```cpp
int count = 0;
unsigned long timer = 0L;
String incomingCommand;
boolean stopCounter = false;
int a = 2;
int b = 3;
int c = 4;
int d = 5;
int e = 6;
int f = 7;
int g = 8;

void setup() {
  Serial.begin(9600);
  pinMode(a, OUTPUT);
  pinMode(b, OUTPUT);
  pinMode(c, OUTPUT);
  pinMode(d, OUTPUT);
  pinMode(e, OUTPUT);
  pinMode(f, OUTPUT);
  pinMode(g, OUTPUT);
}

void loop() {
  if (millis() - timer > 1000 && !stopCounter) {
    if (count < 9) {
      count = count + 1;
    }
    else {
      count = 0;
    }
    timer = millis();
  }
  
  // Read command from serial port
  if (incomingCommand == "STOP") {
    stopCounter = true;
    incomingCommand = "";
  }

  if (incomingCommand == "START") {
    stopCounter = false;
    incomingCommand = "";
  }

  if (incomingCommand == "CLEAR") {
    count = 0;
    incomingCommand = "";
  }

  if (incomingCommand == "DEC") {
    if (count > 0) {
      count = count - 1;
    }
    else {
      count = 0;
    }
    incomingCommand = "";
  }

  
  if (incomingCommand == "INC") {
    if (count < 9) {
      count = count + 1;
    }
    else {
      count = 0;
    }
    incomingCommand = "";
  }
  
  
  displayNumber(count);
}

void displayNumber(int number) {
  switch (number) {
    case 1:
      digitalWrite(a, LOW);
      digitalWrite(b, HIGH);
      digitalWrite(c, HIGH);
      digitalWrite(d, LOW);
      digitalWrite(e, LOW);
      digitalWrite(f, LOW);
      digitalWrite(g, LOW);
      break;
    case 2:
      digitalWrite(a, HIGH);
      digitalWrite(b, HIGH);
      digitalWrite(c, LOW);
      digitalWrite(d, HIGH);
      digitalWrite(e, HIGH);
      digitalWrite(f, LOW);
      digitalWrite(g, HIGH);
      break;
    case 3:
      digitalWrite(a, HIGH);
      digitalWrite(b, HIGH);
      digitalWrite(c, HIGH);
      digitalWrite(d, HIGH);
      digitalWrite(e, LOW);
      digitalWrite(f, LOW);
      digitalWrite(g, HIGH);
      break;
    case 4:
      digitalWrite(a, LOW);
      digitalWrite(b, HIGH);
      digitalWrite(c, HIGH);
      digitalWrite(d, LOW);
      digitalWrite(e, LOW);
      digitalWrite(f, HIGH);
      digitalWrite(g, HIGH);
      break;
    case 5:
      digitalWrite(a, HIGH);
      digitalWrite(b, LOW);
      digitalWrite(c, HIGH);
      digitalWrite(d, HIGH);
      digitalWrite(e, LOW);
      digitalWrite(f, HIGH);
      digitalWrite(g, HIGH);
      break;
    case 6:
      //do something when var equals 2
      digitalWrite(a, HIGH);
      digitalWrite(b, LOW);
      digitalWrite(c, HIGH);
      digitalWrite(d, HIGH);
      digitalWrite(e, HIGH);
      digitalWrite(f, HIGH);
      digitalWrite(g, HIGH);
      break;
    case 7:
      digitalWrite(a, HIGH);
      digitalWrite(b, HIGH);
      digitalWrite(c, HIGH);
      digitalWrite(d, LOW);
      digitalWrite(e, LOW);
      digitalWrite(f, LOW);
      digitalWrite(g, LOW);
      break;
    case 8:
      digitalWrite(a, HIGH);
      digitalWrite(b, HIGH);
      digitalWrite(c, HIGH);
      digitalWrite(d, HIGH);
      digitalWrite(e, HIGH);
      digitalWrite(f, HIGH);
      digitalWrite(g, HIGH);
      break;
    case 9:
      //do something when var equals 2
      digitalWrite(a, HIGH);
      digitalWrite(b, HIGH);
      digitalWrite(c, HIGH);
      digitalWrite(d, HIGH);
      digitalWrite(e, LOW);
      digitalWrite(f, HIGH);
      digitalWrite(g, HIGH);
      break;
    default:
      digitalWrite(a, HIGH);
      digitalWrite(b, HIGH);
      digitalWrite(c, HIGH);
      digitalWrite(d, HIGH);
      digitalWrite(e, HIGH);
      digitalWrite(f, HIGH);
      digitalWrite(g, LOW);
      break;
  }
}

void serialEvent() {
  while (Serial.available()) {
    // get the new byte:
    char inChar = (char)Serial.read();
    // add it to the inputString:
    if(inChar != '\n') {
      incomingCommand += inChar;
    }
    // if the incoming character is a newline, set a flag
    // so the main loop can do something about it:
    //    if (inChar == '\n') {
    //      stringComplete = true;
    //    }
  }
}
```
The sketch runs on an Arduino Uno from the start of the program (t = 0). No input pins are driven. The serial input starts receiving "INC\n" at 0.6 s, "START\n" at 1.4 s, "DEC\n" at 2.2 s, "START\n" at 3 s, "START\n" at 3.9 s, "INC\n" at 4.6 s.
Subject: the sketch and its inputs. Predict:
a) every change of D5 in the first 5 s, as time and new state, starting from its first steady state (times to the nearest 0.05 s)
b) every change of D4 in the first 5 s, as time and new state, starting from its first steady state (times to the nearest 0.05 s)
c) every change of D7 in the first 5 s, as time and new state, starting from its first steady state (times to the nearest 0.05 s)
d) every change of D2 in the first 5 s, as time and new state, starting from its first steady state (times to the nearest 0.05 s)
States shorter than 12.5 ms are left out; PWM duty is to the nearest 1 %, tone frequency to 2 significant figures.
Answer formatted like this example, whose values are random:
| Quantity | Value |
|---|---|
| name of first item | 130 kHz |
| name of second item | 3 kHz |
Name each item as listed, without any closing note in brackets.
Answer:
| Quantity | Value |
|---|---|
| every change of D5 in the first 5 s, as time and new state, starting from its first steady state | 0 s high; 0.6 s low; 1 s high; 4 s low; 4.6 s high |
| every change of D4 in the first 5 s, as time and new state, starting from its first steady state | 0 s high; 1 s low; 2 s high; 2.2 s low; 3 s high |
| every change of D7 in the first 5 s, as time and new state, starting from its first steady state | 0 s high; 0.6 s low; 4 s high |
| every change of D2 in the first 5 s, as time and new state, starting from its first steady state | 0 s high; 0.6 s low; 1 s high; 4 s low; 4.6 s high |
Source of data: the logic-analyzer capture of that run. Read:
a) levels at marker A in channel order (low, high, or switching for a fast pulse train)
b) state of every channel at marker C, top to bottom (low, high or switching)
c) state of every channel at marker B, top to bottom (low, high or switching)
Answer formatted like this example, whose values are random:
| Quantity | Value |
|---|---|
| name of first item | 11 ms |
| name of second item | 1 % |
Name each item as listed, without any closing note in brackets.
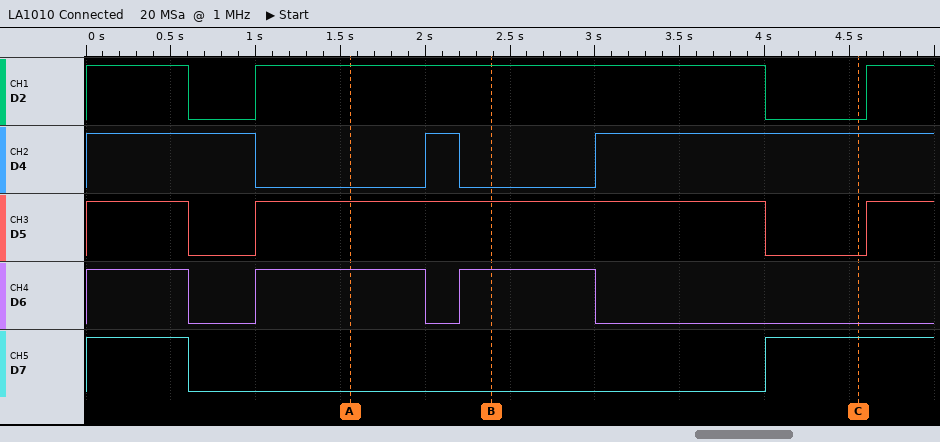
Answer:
| Quantity | Value |
|---|---|
| levels at marker A in channel order | D2 high, D4 low, D5 high, D6 high, D7 low |
| state of every channel at marker C, top to bottom | D2 low, D4 high, D5 low, D6 low, D7 high |
| state of every channel at marker B, top to bottom | D2 high, D4 low, D5 high, D6 high, D7 low |
